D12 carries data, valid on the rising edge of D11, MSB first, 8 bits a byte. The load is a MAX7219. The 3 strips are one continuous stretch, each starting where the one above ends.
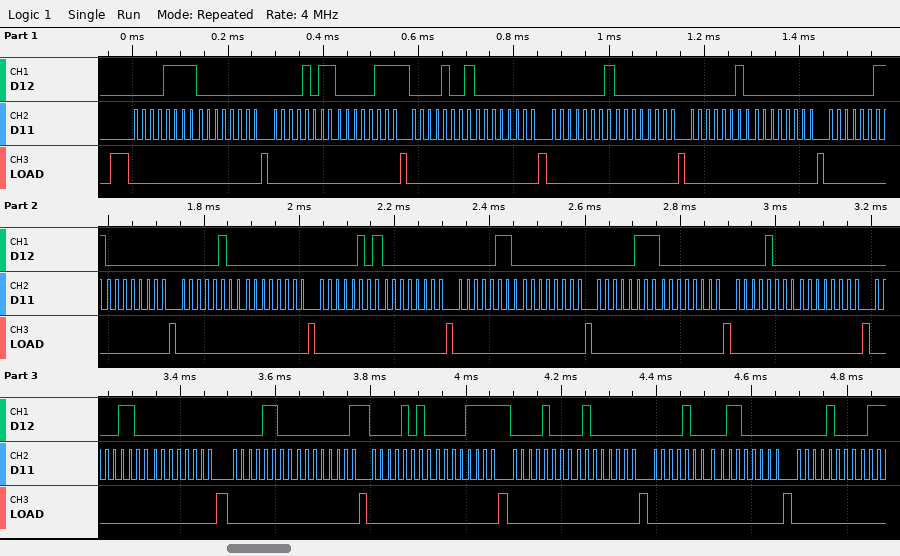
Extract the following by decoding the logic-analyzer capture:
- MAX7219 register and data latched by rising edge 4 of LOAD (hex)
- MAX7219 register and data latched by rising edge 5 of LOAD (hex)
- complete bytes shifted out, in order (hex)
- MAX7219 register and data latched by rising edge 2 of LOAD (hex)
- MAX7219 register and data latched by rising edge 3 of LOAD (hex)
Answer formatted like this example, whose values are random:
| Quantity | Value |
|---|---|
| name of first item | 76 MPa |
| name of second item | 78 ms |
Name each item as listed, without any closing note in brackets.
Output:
| Quantity | Value |
|---|---|
| MAX7219 register and data latched by rising edge 4 of LOAD | register 0x9, data 0x00 |
| MAX7219 register and data latched by rising edge 5 of LOAD | register 0x1, data 0x00 |
| complete bytes shifted out, in order | 0F 00 0B 07 09 00 01 00 02 00 03 00 04 00 05 00 06 00 07 00 08 00 0C 00 0C 01 0A 0F 08 40 08 60 08 |
| MAX7219 register and data latched by rising edge 2 of LOAD | register 0xF, data 0x00 |
| MAX7219 register and data latched by rising edge 3 of LOAD | register 0xB, data 0x07 |
